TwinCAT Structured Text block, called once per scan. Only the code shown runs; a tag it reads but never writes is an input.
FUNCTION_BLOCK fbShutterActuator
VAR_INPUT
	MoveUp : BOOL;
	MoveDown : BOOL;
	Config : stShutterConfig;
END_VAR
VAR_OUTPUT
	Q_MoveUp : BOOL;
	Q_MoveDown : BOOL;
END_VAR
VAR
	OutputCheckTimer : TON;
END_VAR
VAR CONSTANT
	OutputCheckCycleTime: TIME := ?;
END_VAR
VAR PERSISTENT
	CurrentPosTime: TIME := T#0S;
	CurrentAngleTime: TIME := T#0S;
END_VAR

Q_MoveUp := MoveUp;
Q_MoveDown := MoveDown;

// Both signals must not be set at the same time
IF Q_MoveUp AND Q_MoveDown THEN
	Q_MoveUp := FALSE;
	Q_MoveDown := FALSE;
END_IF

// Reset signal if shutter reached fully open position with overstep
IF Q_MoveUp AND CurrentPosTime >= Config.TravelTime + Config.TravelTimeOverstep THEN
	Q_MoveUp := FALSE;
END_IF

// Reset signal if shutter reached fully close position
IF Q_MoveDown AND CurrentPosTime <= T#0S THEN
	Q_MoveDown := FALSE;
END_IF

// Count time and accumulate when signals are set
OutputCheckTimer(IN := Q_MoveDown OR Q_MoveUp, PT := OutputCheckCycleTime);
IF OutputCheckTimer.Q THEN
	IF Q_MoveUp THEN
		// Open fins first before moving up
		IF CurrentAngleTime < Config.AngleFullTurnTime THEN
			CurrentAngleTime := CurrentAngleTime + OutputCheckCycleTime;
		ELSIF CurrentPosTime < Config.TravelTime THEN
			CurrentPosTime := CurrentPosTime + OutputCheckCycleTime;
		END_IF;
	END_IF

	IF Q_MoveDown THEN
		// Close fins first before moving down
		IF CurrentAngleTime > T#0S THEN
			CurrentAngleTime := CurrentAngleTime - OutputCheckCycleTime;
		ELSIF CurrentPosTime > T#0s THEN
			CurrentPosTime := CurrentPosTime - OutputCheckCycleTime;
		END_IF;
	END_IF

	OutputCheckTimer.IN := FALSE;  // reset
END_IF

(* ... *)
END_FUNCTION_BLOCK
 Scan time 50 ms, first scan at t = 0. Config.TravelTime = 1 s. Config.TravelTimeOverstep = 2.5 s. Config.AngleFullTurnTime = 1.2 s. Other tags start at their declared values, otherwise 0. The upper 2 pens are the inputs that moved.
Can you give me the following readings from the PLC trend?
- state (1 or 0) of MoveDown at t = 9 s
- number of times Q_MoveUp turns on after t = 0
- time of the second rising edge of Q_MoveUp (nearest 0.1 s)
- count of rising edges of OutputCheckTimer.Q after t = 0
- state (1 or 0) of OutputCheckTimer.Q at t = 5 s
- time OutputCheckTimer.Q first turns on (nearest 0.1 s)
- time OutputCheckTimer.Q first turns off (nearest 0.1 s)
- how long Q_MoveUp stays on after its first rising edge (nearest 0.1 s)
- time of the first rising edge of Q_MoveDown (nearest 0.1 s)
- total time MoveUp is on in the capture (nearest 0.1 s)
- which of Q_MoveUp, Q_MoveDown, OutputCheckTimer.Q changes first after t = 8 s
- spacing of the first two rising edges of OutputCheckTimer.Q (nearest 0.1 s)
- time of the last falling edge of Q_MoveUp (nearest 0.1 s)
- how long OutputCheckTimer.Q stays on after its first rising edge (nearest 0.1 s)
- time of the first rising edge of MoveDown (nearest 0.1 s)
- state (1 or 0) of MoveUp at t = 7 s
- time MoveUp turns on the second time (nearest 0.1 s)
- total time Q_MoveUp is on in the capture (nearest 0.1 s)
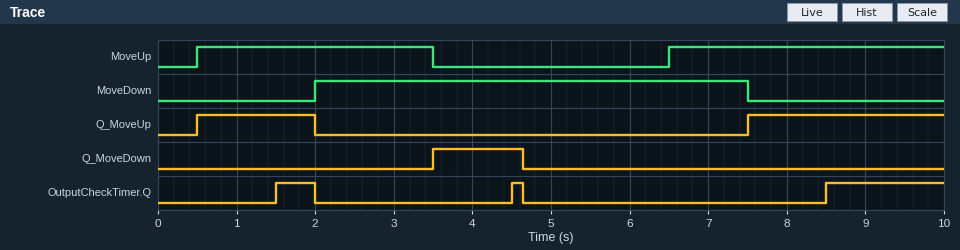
0
2
7.5 s
3
0
1.5 s
2.0 s
1.5 s
3.5 s
6.5 s
OutputCheckTimer.Q
3.0 s
2.0 s
0.5 s
2.0 s
1
6.5 s
4.0 s
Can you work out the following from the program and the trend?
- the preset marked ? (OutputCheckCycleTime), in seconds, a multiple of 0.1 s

1.0 s
